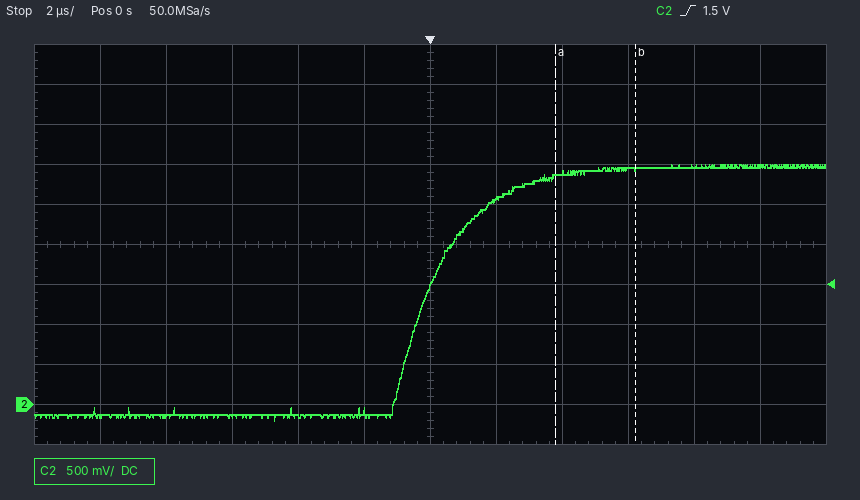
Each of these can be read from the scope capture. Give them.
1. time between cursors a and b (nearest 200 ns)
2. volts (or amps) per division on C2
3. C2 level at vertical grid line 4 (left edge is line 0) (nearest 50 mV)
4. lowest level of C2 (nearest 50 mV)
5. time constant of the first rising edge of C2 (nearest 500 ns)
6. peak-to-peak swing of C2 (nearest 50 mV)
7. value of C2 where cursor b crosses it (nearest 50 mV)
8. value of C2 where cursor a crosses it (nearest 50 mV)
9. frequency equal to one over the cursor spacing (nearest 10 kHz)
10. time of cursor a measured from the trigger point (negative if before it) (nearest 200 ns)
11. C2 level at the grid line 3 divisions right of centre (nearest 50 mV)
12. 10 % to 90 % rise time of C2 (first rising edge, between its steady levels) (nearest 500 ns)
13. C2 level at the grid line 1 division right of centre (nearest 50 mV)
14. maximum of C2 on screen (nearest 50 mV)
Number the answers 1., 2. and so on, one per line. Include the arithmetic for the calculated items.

1. 2.4 µs
2. 500 mV
3. -150 mV
4. -200 mV
5. 3.5 µs / 2.2 ≈ 1.59 µs, so 1.5 µs to the nearest 500 ns
6. 3.00 V − (-200 mV) = 3.20 V
7. 2.95 V
8. 2.85 V
9. 1 / 2.4 µs ≈ 420 kHz
10. +3.8 µs
11. 2.95 V
12. 3.5 µs
13. 2.55 V
14. 3.00 V
